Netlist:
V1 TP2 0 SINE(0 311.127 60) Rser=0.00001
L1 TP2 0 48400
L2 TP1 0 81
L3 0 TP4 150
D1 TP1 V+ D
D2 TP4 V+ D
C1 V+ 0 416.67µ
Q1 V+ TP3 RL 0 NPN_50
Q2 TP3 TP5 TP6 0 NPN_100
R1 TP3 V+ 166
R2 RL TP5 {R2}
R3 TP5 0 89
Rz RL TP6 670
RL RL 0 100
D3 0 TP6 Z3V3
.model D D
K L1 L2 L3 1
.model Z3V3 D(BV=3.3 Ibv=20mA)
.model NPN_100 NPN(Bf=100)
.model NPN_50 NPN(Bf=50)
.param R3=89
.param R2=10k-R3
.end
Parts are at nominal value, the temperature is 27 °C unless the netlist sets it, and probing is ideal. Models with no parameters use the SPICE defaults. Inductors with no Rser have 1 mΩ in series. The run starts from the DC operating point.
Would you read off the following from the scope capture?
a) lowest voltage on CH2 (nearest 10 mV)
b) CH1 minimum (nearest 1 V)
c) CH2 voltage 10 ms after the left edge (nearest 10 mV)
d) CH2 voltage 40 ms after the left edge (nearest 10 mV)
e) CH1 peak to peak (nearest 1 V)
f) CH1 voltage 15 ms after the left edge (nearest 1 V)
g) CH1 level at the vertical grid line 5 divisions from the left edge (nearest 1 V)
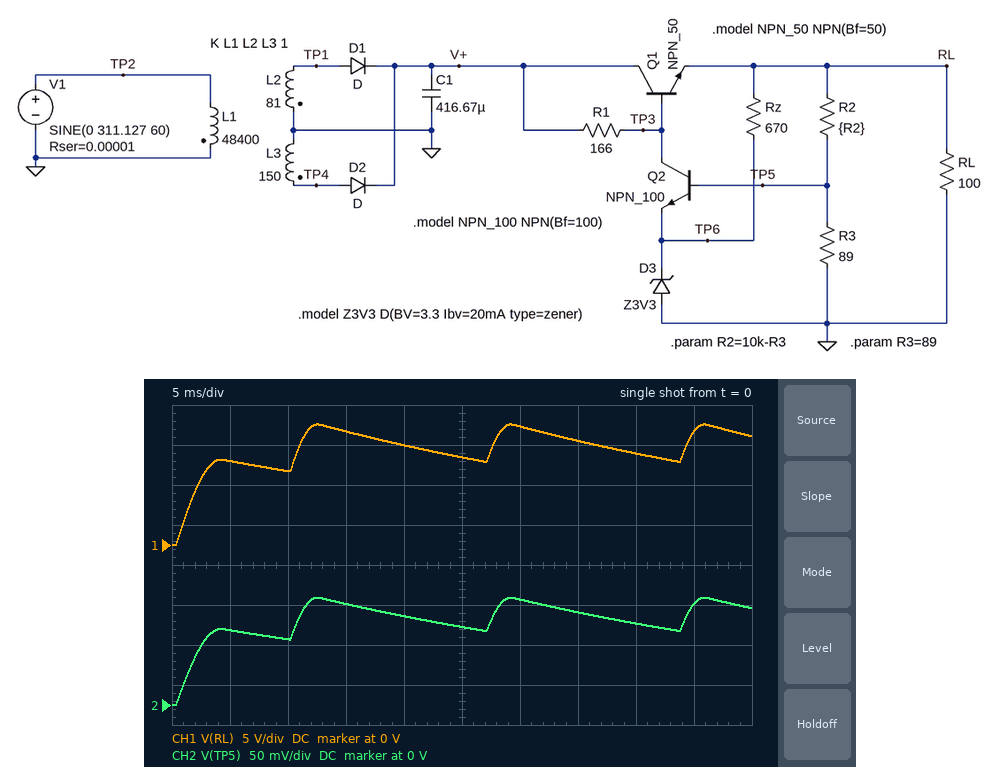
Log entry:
0 V
0 V
80 mV
100 mV
15 V
14 V
11 V
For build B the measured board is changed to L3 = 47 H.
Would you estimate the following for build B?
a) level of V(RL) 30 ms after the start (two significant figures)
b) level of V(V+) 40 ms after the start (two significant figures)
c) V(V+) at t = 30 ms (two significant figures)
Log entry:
8.5 V
11 V
9.7 V
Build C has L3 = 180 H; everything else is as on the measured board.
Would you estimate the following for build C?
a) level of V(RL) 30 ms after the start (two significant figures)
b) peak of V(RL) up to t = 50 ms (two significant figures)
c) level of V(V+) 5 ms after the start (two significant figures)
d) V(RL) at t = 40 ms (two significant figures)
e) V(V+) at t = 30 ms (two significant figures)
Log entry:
16 V
17 V
12 V
13 V
18 V
